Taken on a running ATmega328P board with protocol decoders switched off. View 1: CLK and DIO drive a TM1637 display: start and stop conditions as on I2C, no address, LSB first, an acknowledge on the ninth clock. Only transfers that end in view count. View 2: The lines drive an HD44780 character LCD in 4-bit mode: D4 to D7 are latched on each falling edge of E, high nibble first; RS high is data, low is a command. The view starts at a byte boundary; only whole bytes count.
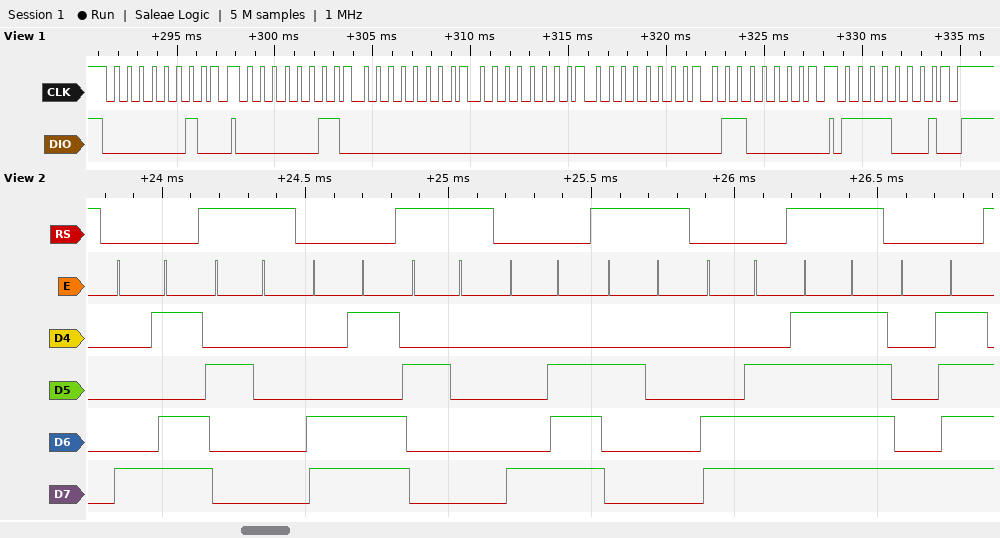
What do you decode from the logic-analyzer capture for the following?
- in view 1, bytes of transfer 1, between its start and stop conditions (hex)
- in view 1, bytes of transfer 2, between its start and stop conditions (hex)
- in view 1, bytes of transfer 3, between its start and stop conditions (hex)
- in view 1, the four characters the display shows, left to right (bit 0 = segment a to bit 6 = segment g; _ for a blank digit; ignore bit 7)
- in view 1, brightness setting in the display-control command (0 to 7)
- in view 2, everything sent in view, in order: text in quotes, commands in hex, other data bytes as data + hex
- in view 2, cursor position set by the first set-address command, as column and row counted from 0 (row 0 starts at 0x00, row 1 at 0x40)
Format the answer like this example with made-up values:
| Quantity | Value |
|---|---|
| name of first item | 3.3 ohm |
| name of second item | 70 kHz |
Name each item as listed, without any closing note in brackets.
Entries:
| Quantity | Value |
|---|---|
| in view 1, bytes of transfer 1, between its start and stop conditions | 40 |
| in view 1, bytes of transfer 2, between its start and stop conditions | C0 00 00 00 06 |
| in view 1, bytes of transfer 3, between its start and stop conditions | 8F |
| in view 1, the four characters the display shows, left to right | ___1 |
| in view 1, brightness setting in the display-control command | 7 |
| in view 2, everything sent in view, in order: text in quotes, commands in hex, other data bytes as data + hex | 0x8D " " 0xCD " " 0x8E " " 0xCE data FF 0x8F |
| in view 2, cursor position set by the first set-address command, as column and row counted from 0 | column 13, row 0 |
